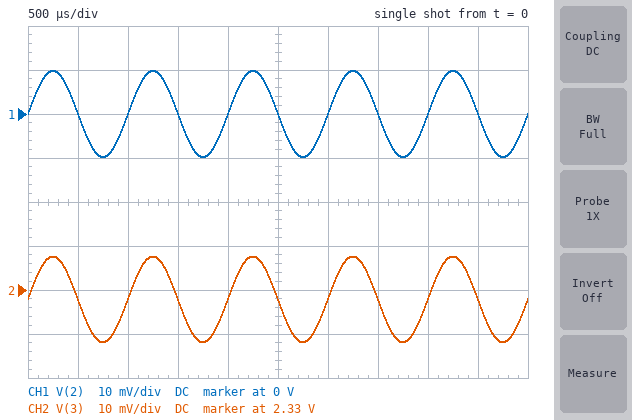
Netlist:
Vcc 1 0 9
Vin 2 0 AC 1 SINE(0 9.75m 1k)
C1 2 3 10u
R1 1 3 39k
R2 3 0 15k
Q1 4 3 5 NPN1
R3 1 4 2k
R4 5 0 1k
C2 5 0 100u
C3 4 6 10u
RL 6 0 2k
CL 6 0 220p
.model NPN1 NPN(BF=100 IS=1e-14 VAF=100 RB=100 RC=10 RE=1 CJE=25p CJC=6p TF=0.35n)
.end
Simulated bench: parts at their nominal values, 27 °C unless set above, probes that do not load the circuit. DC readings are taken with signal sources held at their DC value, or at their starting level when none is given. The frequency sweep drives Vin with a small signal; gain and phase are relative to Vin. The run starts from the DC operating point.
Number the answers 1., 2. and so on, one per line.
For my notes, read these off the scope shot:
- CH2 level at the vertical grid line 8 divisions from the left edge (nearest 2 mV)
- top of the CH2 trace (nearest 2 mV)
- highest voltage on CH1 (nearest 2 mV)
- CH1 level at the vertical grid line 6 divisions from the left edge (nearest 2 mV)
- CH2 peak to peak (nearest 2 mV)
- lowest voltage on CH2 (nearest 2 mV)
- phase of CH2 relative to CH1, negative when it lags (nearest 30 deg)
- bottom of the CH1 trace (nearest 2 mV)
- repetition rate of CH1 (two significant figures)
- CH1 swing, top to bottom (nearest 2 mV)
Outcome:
1. 2.328 V
2. 2.338 V
3. 10 mV
4. 0 V
5. 20 mV
6. 2.318 V
7. 0 deg
8. -10 mV
9. 1.0 kHz
10. 20 mV
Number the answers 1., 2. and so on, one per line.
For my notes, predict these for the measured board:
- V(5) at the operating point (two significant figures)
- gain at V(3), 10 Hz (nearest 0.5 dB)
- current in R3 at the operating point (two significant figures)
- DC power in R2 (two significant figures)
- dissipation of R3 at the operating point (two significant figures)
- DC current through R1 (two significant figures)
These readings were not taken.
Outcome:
1. 1.7 V
2. -1.0 dB
3. 1.6 mA
4. 360 µW
5. 5.4 mW
6. 170 µA
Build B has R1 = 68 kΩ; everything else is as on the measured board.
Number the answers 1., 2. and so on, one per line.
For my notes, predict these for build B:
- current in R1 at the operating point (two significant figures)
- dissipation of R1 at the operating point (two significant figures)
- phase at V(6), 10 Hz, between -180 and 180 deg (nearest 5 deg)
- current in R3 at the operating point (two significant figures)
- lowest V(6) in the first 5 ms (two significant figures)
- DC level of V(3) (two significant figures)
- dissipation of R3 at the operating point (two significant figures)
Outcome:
1. 110 µA
2. 820 µW
3. -80 deg
4. 870 µA
5. -330 mV
6. 1.5 V
7. 1.5 mW
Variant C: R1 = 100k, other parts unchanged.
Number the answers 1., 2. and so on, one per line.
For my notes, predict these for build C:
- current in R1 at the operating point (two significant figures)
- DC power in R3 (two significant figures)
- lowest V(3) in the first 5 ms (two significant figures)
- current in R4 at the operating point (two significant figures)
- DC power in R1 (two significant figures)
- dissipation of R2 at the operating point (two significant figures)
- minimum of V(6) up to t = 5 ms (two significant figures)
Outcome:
1. 79 µA
2. 450 µW
3. 1.1 V
4. 480 µA
5. 620 µW
6. 83 µW
7. -200 mV
